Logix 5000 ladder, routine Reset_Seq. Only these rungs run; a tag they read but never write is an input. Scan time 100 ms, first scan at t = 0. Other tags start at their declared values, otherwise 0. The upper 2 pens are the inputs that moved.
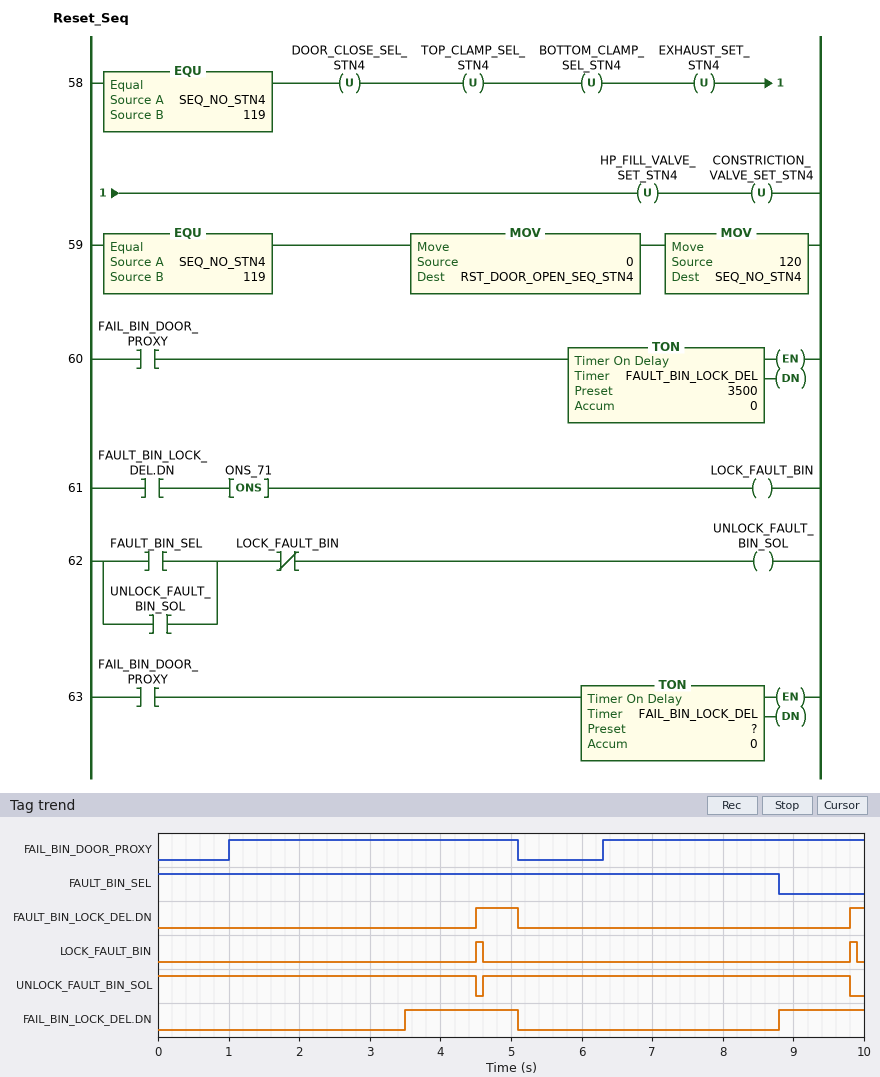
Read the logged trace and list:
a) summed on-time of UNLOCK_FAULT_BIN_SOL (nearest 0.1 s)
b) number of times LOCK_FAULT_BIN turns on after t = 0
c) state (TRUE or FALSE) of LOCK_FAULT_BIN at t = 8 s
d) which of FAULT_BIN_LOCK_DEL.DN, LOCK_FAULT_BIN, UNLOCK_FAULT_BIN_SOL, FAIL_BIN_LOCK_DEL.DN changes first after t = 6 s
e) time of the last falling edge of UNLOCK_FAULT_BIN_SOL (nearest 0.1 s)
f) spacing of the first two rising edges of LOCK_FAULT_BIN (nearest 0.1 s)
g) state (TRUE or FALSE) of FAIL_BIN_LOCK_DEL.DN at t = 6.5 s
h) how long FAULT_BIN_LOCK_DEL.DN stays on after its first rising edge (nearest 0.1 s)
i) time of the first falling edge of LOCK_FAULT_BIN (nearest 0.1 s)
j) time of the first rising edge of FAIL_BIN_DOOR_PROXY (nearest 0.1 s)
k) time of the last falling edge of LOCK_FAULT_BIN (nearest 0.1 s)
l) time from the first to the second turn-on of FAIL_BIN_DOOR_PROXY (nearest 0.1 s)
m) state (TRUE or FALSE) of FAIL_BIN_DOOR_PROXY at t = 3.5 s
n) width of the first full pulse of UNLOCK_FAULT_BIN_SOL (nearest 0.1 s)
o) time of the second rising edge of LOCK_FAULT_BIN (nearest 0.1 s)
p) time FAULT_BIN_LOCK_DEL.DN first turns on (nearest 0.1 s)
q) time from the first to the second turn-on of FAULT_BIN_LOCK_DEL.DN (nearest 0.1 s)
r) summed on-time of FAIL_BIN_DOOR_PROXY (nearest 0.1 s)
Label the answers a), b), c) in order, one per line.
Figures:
a) 9.7 s
b) 2
c) FALSE
d) FAIL_BIN_LOCK_DEL.DN
e) 9.8 s
f) 5.3 s
g) FALSE
h) 0.6 s
i) 4.6 s
j) 1.0 s
k) 9.9 s
l) 5.3 s
m) TRUE
n) 5.2 s
o) 9.8 s
p) 4.5 s
q) 5.3 s
r) 7.8 s
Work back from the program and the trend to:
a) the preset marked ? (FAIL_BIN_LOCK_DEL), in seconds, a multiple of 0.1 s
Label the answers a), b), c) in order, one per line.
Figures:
a) 2.5 s
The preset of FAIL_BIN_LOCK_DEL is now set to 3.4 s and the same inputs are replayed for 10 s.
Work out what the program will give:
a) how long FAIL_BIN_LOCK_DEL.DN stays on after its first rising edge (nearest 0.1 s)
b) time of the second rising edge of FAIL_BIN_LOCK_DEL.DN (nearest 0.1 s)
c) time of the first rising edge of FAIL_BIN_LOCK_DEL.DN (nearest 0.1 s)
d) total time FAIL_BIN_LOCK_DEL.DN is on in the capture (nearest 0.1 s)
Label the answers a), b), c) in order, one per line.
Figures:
a) 0.7 s
b) 9.7 s
c) 4.4 s
d) 1.0 s
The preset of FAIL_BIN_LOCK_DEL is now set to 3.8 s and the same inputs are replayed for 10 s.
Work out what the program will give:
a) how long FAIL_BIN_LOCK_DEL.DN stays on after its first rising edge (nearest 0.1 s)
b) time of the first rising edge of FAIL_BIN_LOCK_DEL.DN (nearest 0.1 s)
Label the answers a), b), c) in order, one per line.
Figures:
a) 0.3 s
b) 4.8 s
